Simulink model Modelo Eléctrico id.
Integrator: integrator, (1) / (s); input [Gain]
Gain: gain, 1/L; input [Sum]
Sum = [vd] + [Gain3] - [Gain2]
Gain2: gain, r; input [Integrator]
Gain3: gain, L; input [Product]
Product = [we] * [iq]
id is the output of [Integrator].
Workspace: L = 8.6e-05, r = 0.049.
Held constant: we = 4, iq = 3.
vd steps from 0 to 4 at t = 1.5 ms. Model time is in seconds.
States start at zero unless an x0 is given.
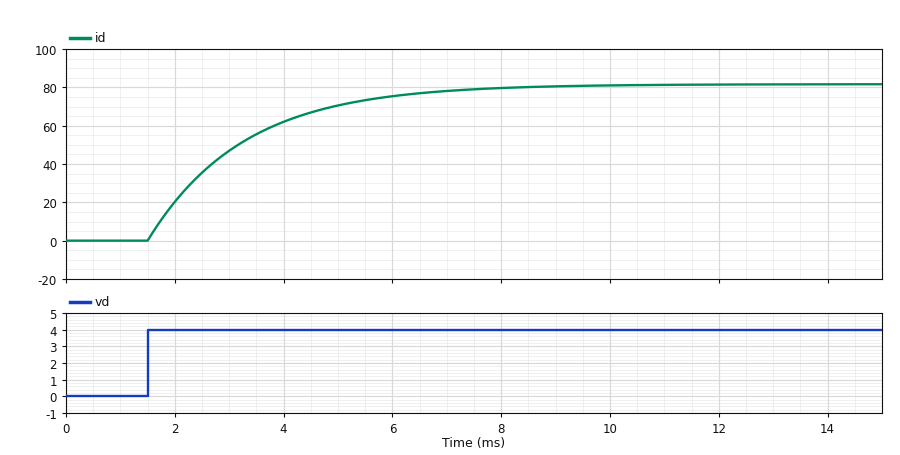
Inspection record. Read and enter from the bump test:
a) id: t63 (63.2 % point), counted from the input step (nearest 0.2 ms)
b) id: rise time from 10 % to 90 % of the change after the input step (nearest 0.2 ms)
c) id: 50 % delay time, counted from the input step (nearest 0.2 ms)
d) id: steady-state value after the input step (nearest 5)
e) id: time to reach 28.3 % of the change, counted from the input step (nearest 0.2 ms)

1.8 ms
3.8 ms
1.2 ms
80
0.6 ms
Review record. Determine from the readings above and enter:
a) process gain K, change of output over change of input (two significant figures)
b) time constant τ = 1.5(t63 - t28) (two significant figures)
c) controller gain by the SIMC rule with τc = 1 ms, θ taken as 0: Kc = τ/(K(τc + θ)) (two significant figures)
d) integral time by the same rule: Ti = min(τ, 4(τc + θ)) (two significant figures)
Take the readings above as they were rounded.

20
1.8 ms
0.090
1.8 ms
